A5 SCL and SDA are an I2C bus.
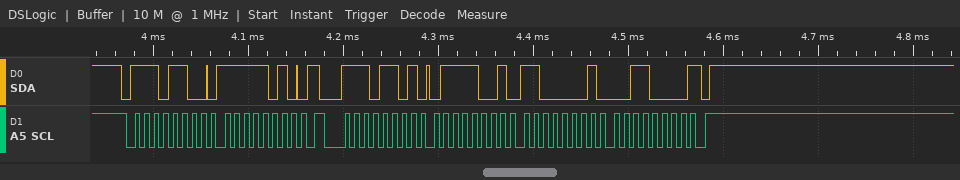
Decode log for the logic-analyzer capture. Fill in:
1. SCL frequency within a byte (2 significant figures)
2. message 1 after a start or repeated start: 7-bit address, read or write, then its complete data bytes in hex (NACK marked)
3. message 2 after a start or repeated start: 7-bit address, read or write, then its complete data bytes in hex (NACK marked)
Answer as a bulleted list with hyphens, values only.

- 100 kHz
- 0x76 write: FA
- 0x76 read: 79 C1 30 NACK
